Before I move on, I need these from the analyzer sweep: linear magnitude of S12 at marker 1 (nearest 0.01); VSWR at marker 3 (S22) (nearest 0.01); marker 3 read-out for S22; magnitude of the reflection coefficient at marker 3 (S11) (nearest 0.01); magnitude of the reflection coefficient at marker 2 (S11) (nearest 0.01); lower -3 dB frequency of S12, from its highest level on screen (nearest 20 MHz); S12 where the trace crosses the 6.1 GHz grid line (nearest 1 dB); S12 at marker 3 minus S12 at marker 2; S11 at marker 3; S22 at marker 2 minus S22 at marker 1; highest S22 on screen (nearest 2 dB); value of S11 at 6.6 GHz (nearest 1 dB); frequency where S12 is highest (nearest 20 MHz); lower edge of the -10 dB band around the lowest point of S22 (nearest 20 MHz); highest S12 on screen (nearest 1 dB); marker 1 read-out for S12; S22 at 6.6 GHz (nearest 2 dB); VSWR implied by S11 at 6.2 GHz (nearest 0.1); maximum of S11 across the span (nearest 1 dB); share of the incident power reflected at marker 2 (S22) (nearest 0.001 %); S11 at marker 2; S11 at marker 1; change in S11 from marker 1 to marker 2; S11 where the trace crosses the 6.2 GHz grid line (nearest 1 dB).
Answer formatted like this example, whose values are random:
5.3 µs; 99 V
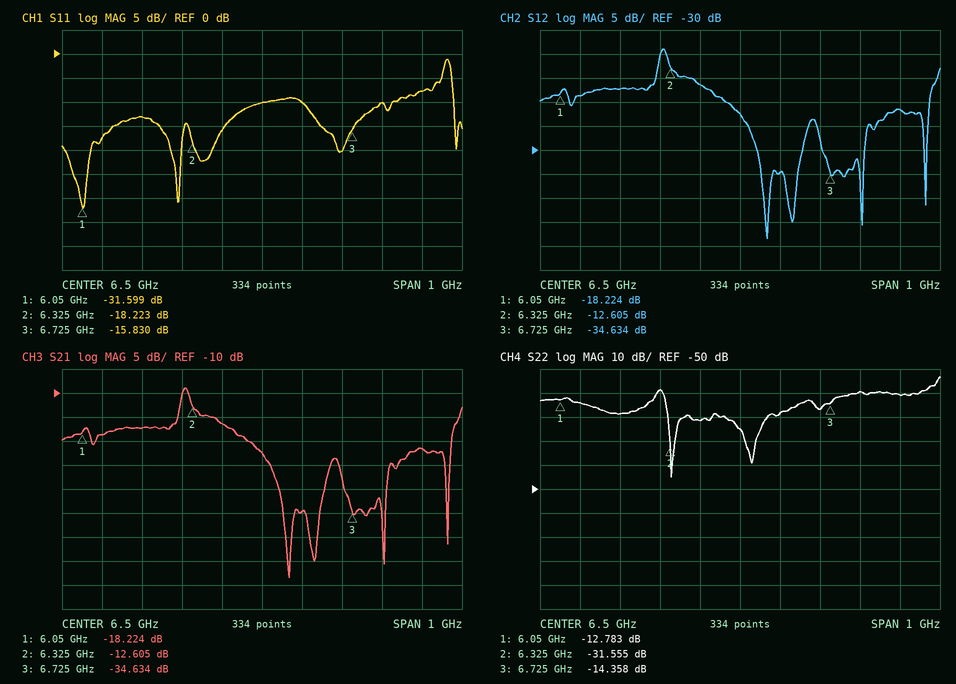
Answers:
0.12; 1.47; -14.358 dB; 0.16; 0.12; 6.30 GHz; -19 dB; -22.029 dB; -15.830 dB; -18.772 dB; -4 dB; -10 dB; 6.30 GHz; 6.30 GHz; -9 dB; -18.224 dB; -18 dB; 1.6; -1 dB; 0.070 %; -18.223 dB; -31.599 dB; 13.376 dB; -13 dB
